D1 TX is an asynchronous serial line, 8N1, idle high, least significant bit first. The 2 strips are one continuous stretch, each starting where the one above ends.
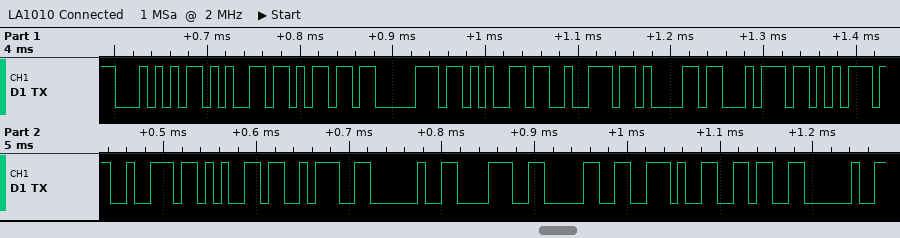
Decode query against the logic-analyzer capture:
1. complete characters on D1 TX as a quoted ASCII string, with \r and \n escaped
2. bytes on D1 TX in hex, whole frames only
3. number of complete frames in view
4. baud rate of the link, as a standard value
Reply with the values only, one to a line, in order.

"Temperature: 80.6 "
54 65 6D 70 65 72 61 74 75 72 65 3A 20 38 30 2E 36 20
18
115200 baud
